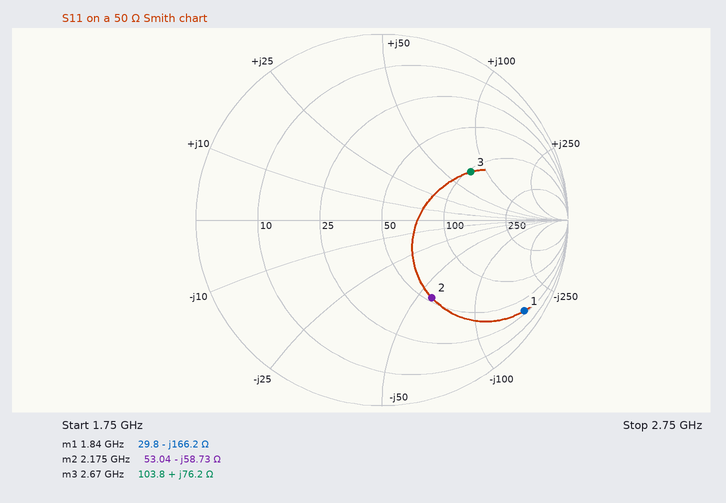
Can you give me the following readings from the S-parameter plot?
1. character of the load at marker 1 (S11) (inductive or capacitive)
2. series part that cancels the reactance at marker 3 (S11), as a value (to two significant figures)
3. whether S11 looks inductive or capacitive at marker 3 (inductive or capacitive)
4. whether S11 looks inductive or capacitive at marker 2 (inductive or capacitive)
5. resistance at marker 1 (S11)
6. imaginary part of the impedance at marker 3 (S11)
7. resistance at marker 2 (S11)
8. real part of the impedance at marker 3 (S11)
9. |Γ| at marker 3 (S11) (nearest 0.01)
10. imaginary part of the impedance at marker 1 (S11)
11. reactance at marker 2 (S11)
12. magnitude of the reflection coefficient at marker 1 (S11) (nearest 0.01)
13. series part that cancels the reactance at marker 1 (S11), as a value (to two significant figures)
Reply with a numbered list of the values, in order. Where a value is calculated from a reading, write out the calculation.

1. capacitive
2. C = 1/(2π × 2.67 GHz × 76.2 Ω) ≈ 782 fF, so 780 fF to two significant figures
3. inductive
4. capacitive
5. 29.8 Ω
6. +76.2 Ω
7. 53.04 Ω
8. 103.8 Ω
9. 0.54
10. -166.2 Ω
11. -58.73 Ω
12. 0.91
13. L = 166.2 Ω/(2π × 1.84 GHz) ≈ 14 nH
